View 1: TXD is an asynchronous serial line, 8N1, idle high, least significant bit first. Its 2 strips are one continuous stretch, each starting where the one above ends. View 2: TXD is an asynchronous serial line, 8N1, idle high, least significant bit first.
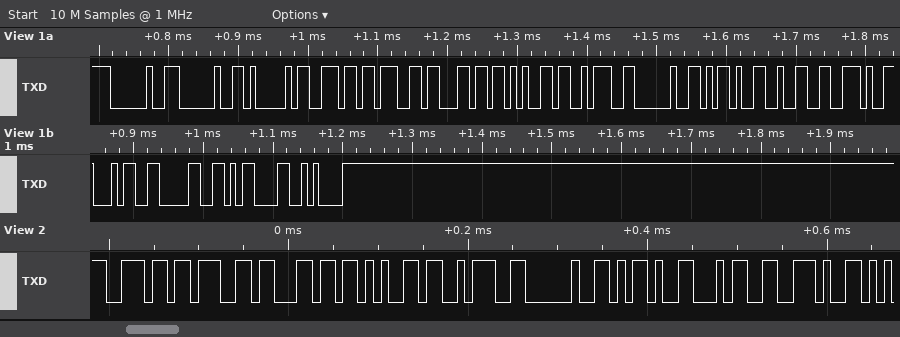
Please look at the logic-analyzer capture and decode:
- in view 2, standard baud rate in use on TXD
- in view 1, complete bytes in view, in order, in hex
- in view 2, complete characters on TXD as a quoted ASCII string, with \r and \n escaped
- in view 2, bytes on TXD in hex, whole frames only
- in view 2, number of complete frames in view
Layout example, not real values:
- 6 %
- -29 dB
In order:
- 115200 baud
- 20 20 41 6E 67 6C 65 3A 20 2D 32 2E 34 30 0D 0A
- "ngle: -4."
- 0x6E 0x67 0x6C 0x65 0x3A 0x20 0x2D 0x34 0x2E
- 9
